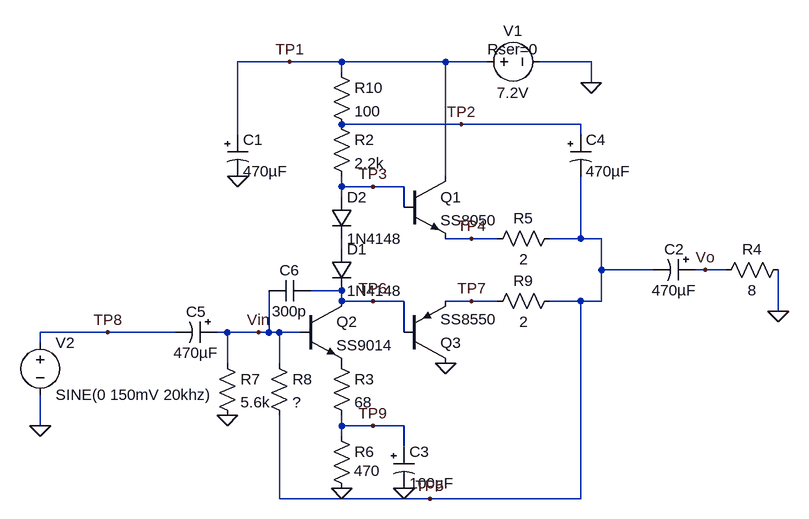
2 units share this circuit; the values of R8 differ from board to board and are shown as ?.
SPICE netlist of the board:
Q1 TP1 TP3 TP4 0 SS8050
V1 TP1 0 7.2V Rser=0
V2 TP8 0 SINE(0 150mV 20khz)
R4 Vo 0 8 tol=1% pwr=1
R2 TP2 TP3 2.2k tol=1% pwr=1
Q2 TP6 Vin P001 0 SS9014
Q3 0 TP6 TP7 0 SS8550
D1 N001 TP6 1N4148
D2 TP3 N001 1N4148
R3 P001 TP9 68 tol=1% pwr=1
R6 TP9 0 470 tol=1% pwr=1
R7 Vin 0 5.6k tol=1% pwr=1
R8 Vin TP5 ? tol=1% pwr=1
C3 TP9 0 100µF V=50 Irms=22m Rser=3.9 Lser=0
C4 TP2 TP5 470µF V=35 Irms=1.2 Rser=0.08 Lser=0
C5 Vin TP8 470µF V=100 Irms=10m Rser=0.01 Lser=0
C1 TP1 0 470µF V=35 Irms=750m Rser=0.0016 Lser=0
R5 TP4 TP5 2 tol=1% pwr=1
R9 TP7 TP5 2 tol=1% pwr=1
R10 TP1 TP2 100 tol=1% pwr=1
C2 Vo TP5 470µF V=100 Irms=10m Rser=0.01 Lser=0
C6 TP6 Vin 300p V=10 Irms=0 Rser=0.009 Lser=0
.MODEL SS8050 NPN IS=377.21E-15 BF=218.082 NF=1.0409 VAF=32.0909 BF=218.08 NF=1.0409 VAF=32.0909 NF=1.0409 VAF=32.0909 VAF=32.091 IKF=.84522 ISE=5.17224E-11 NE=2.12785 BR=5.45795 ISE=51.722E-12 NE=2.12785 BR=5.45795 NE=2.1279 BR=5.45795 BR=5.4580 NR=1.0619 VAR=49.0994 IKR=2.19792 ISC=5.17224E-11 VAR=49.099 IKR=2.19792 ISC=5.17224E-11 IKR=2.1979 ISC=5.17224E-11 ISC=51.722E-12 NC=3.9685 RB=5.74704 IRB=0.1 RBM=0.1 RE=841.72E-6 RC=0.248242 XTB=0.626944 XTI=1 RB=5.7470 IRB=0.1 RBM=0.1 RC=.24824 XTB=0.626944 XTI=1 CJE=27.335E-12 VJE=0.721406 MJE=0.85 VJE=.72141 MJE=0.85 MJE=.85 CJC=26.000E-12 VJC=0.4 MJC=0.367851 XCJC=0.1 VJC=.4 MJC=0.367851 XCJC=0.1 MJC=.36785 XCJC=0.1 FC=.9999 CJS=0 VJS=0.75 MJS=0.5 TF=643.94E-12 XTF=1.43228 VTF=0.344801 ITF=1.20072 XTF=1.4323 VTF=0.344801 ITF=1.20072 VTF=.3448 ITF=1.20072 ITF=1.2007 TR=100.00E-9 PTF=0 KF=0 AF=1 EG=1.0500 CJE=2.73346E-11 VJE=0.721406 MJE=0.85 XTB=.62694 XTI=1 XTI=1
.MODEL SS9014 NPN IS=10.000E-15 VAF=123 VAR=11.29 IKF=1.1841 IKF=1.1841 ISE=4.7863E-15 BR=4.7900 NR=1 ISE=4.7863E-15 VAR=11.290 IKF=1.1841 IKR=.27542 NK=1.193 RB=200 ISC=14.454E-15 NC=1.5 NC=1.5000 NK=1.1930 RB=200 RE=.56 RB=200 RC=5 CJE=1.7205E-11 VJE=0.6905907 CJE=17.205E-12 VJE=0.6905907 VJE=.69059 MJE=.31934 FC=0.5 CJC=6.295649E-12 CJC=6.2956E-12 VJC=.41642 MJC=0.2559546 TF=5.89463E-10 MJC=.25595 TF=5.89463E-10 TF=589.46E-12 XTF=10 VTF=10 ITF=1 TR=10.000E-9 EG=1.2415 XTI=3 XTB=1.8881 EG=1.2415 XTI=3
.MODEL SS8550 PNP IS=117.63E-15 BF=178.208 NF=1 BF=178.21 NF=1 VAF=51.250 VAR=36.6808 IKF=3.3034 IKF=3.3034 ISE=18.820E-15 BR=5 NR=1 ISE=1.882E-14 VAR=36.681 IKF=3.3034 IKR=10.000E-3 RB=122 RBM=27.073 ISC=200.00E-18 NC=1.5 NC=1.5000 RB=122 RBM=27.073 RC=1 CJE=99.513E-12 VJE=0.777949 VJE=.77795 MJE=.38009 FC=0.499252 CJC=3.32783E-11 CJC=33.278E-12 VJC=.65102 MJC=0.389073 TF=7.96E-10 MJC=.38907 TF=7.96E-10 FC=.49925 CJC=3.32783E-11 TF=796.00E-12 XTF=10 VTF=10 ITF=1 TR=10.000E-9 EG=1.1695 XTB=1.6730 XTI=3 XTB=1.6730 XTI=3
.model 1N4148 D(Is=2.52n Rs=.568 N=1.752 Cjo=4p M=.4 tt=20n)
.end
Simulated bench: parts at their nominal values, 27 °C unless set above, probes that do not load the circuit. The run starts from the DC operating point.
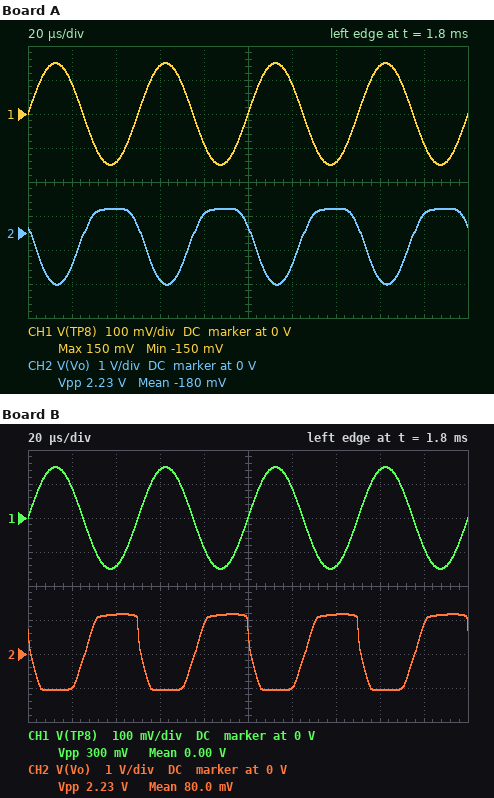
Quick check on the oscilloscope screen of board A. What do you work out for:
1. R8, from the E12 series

22 kΩ
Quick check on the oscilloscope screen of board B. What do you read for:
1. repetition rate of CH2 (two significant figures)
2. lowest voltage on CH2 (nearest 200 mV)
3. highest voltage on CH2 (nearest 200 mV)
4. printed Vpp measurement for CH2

20 kHz
-1.0 V
1.2 V
2.23 V
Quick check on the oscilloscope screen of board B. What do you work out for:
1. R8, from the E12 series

5.6 kΩ
